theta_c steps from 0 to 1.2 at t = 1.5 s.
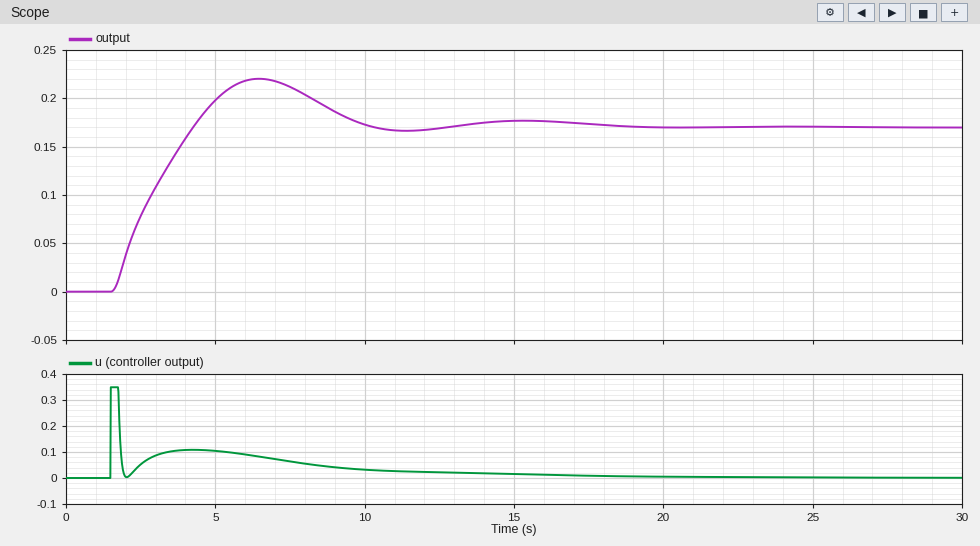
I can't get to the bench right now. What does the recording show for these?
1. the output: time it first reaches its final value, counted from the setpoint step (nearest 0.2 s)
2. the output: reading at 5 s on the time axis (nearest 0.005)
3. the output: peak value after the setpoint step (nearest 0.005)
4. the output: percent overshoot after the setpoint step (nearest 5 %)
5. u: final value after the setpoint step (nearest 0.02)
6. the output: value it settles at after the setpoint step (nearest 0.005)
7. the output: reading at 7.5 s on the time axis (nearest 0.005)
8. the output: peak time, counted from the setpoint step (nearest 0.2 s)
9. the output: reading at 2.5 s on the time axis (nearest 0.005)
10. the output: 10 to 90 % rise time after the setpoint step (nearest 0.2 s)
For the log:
2.8 s
0.200
0.220
30 %
0.00
0.170
0.210
5.0 s
0.080
2.0 s
